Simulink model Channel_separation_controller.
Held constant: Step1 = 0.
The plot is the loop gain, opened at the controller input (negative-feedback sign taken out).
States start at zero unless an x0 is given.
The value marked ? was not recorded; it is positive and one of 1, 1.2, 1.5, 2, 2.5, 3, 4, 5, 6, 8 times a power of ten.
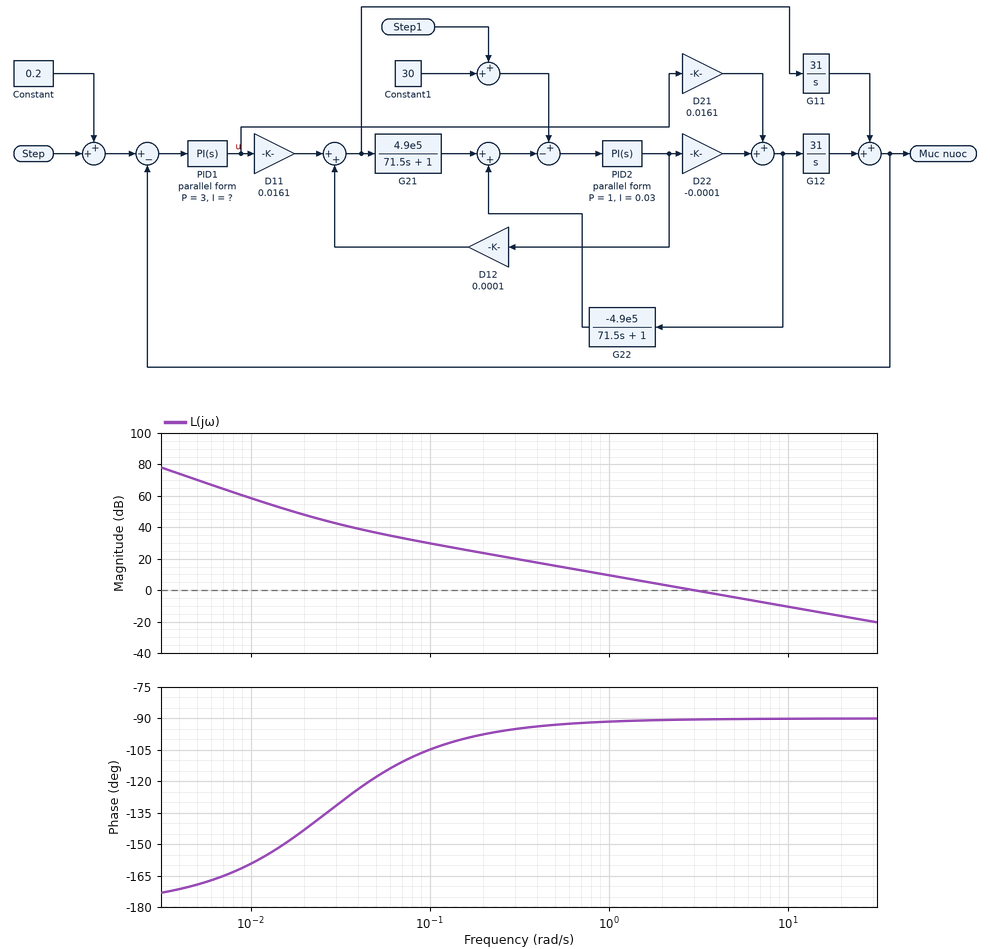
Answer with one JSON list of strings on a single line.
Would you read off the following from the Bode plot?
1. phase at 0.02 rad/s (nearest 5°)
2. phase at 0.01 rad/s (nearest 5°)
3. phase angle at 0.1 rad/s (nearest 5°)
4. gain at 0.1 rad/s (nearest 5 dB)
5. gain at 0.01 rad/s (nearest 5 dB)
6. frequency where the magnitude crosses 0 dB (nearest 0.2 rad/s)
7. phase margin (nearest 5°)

["-145°", "-160°", "-105°", "30 dB", "60 dB", "3.0 rad/s", "90°"]
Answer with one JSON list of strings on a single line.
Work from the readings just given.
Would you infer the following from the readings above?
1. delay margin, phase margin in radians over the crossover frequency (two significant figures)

["0.52 s"]
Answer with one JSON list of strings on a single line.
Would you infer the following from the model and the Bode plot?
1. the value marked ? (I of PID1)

["0.08"]
